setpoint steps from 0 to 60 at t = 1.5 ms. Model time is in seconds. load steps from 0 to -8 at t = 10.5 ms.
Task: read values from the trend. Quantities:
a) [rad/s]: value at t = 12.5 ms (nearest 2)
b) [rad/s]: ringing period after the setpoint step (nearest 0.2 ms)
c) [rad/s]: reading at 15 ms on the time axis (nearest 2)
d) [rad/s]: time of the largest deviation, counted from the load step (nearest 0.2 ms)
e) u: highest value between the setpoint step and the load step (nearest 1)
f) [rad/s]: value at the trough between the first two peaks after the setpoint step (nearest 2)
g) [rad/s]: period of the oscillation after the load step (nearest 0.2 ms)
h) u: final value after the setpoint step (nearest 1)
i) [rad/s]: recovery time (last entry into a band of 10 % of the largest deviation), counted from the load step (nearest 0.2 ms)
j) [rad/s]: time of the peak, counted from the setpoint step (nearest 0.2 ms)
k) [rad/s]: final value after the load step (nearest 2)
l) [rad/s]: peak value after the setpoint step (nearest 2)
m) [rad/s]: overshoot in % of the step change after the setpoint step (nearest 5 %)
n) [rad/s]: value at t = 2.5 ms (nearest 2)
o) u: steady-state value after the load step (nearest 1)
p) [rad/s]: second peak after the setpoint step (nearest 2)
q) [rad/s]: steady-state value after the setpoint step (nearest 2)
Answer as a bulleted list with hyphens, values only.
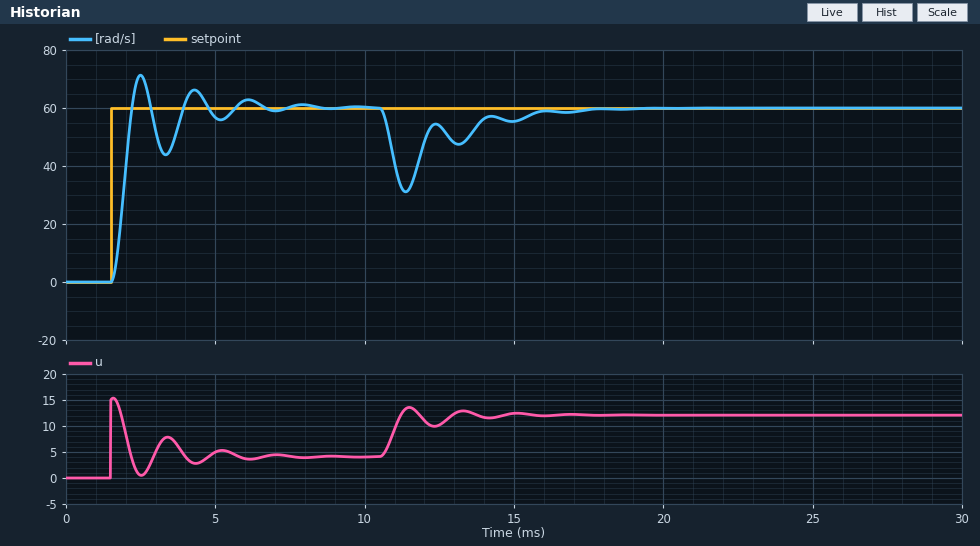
- 54
- 1.8 ms
- 56
- 0.8 ms
- 15
- 44
- 1.8 ms
- 4
- 5.0 ms
- 1.0 ms
- 60
- 72
- 20 %
- 72
- 12
- 66
- 60
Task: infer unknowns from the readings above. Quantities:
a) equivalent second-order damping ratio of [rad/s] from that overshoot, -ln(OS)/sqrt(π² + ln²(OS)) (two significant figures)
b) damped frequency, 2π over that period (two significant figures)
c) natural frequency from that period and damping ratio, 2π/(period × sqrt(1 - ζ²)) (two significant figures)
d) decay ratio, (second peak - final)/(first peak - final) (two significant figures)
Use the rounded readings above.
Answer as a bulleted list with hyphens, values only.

- 0.46
- 3.5 rad/ms
- 3.9 rad/ms
- 0.50
